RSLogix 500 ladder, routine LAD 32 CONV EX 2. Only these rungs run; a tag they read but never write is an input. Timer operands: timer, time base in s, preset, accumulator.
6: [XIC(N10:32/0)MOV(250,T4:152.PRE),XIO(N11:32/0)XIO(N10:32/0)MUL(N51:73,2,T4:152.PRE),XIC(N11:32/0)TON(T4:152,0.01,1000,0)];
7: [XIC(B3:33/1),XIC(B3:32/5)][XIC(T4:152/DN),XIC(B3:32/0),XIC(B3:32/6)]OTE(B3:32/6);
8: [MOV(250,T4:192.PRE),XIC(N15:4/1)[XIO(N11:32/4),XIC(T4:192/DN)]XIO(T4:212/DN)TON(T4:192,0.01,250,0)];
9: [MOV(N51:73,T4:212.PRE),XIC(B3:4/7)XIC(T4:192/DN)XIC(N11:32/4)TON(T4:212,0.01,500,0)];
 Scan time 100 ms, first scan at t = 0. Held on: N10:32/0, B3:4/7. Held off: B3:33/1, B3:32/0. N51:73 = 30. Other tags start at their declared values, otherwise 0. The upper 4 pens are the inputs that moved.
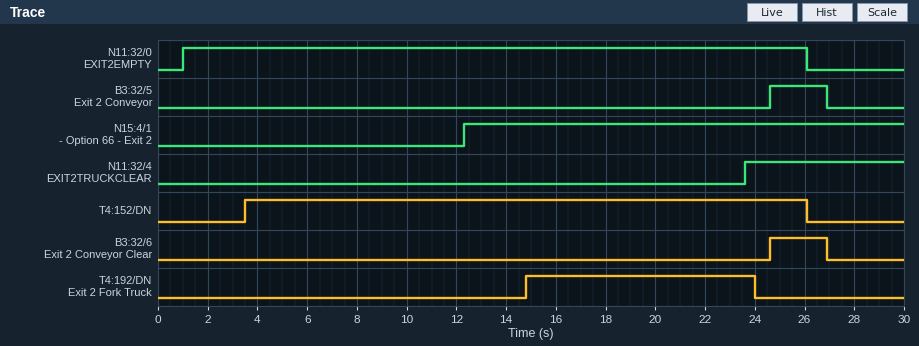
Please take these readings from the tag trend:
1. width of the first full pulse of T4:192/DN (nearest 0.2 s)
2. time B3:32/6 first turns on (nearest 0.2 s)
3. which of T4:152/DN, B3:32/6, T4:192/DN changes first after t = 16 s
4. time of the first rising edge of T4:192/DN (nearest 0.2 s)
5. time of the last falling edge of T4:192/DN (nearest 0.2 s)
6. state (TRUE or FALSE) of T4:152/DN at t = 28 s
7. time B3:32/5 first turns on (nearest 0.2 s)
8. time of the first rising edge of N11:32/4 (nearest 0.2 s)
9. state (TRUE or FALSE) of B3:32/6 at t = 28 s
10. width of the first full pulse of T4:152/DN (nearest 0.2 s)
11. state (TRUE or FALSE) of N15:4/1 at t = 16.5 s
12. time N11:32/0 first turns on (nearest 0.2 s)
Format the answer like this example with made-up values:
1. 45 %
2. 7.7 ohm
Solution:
1. 9.2 s
2. 24.6 s
3. T4:192/DN
4. 14.8 s
5. 24.0 s
6. FALSE
7. 24.6 s
8. 23.6 s
9. FALSE
10. 22.6 s
11. TRUE
12. 1.0 s
